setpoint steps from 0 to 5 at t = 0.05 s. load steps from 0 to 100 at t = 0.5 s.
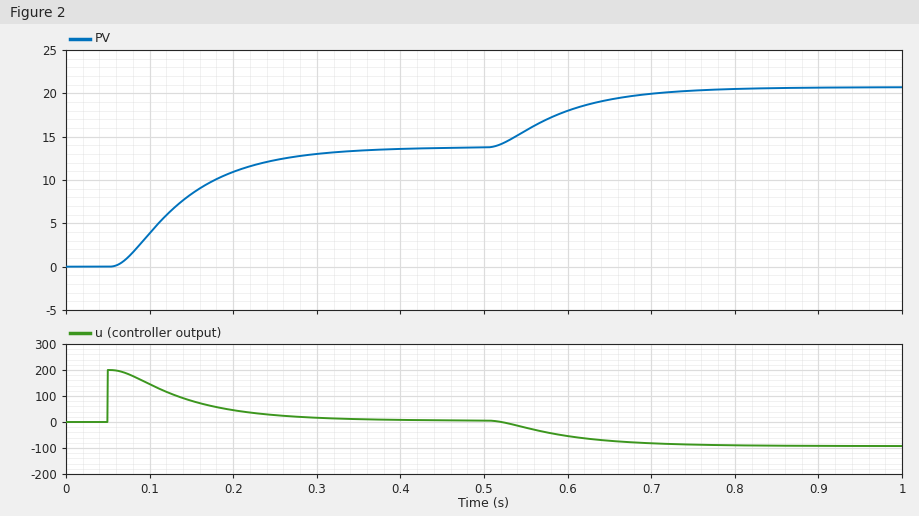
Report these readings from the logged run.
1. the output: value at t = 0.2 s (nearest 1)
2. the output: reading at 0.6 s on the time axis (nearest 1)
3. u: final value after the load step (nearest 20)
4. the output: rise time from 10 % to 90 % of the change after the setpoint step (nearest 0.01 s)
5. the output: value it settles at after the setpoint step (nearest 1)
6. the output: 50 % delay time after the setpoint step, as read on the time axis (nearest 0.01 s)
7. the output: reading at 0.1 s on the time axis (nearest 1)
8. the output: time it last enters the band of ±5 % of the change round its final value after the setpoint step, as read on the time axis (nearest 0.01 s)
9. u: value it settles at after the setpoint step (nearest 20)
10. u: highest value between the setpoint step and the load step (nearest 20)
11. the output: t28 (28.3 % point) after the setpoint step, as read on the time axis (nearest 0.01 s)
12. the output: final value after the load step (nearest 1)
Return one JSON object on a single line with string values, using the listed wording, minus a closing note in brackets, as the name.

{"the output: value at t = 0.2 s": "11", "the output: reading at 0.6 s on the time axis": "18", "u: final value after the load step": "-100", "the output: rise time from 10 % to 90 % of the change after the setpoint step": "0.18 s", "the output: value it settles at after the setpoint step": "14", "the output: 50 % delay time after the setpoint step, as read on the time axis": "0.13 s", "the output: reading at 0.1 s on the time axis": "4", "the output: time it last enters the band of ±5 % of the change round its final value after the setpoint step, as read on the time axis": "0.31 s", "u: value it settles at after the setpoint step": "0", "u: highest value between the setpoint step and the load step": "200", "the output: t28 (28.3 % point) after the setpoint step, as read on the time axis": "0.10 s", "the output: final value after the load step": "21"}
